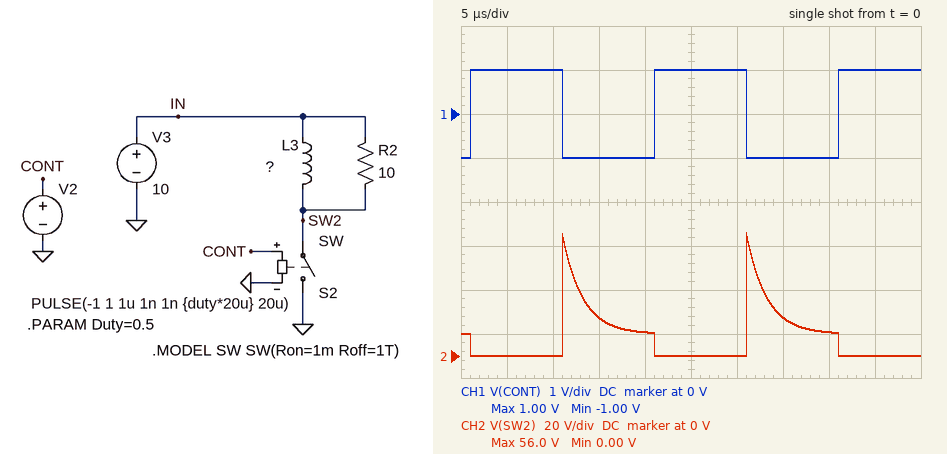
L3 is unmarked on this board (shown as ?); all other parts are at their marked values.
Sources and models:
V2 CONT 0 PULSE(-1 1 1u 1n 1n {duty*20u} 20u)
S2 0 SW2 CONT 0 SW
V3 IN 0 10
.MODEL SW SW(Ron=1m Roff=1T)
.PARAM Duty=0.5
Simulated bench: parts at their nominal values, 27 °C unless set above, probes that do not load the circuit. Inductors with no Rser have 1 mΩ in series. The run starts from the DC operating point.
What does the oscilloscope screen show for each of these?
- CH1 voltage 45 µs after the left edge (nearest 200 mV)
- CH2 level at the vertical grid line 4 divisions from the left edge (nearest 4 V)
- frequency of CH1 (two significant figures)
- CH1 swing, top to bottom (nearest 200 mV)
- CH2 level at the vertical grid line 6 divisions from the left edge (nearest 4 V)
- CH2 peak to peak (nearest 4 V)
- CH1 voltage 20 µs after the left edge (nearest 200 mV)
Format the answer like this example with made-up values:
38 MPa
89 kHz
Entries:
1.0 V
12 V
50 kHz
2.0 V
0 V
56 V
-1.0 V
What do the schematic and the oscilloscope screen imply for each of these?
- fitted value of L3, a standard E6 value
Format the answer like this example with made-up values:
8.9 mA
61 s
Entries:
22 µH
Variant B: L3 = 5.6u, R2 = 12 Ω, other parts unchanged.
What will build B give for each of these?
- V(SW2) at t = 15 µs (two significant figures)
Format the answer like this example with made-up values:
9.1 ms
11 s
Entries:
10 V
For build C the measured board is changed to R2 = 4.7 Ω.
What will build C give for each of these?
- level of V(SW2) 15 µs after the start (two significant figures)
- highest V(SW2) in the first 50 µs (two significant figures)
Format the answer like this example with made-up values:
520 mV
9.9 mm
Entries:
19 V
34 V
